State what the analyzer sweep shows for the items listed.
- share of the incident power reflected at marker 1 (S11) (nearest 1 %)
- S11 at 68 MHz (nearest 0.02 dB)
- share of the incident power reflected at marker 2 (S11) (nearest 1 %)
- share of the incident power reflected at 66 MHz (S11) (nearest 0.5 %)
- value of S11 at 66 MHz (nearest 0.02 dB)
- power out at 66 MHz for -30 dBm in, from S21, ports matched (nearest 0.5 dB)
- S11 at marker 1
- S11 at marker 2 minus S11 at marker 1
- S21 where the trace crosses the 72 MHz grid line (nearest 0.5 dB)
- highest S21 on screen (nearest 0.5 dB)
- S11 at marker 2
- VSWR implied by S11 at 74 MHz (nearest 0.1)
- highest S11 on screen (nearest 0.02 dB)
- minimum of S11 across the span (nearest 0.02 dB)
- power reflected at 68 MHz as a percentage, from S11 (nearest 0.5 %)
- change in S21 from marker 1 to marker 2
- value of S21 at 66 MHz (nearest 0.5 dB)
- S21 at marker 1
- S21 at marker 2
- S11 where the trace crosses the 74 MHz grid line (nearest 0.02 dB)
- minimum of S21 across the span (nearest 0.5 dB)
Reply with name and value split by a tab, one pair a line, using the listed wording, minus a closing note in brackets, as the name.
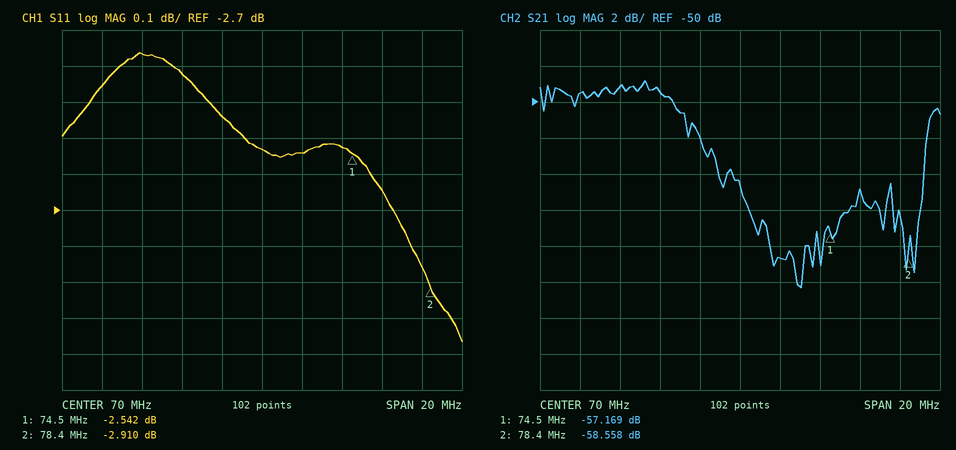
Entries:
share of the incident power reflected at marker 1 (S11)	56 %
S11 at 68 MHz	-2.44 dB
share of the incident power reflected at marker 2 (S11)	51 %
share of the incident power reflected at 66 MHz (S11)	58.5 %
value of S11 at 66 MHz	-2.32 dB
power out at 66 MHz for -30 dBm in, from S21, ports matched	-79.5 dBm
S11 at marker 1	-2.542 dB
S11 at marker 2 minus S11 at marker 1	-0.368 dB
S21 where the trace crosses the 72 MHz grid line	-58.5 dB
highest S21 on screen	-49.0 dB
S11 at marker 2	-2.910 dB
VSWR implied by S11 at 74 MHz	6.9
highest S11 on screen	-2.26 dB
minimum of S11 across the span	-3.06 dB
power reflected at 68 MHz as a percentage, from S11	57.0 %
change in S21 from marker 1 to marker 2	-1.389 dB
value of S21 at 66 MHz	-49.5 dB
S21 at marker 1	-57.169 dB
S21 at marker 2	-58.558 dB
S11 where the trace crosses the 74 MHz grid line	-2.52 dB
minimum of S21 across the span	-60.5 dB
